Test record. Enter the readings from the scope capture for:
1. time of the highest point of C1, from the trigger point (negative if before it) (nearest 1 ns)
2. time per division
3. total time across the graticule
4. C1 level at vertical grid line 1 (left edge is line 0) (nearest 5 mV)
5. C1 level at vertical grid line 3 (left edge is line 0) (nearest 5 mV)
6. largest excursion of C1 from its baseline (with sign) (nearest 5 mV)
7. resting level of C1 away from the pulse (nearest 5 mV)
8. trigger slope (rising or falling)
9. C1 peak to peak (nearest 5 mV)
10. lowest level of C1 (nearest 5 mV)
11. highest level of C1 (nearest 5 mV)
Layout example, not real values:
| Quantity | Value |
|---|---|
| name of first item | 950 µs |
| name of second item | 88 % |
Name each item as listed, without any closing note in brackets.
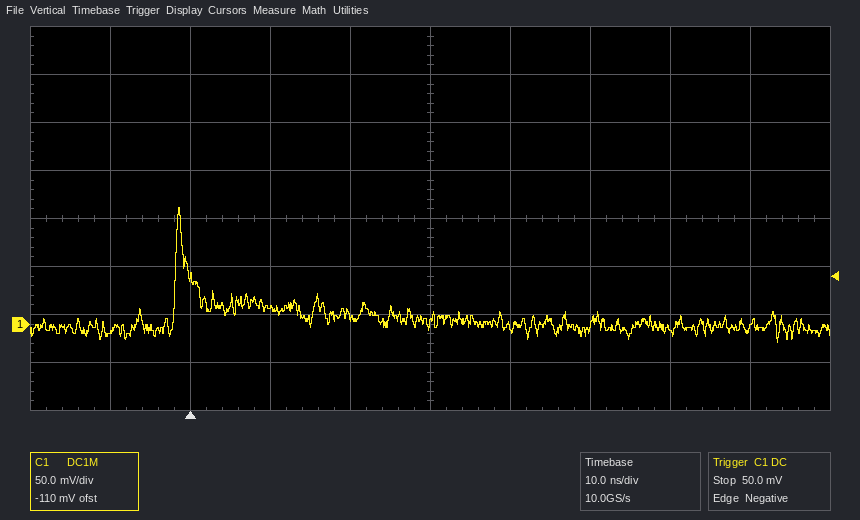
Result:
| Quantity | Value |
|---|---|
| time of the highest point of C1, from the trigger point (negative if before it) | -1 ns |
| time per division | 10 ns |
| total time across the graticule | 100 ns |
| C1 level at vertical grid line 1 (left edge is line 0) | -10 mV |
| C1 level at vertical grid line 3 (left edge is line 0) | 15 mV |
| largest excursion of C1 from its baseline (with sign) | +120 mV |
| resting level of C1 away from the pulse | 0 mV |
| trigger slope | falling |
| C1 peak to peak | 140 mV |
| lowest level of C1 | -20 mV |
| highest level of C1 | 120 mV |
